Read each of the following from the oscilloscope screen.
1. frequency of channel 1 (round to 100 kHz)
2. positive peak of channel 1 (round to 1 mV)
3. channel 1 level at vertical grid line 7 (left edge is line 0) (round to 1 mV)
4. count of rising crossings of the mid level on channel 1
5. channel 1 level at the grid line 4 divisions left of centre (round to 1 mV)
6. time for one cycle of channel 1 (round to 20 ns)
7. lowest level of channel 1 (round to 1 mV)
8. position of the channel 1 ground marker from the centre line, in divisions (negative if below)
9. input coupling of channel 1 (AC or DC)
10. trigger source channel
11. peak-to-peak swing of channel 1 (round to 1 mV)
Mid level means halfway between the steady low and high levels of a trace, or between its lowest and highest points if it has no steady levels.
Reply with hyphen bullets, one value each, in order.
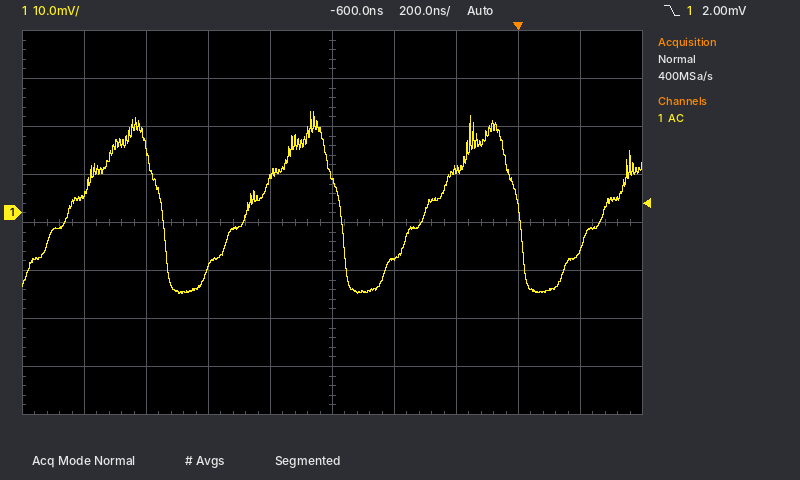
- 1.7 MHz
- 21 mV
- 9 mV
- 4
- 4 mV
- 580 ns
- -17 mV
- +0.2 div
- AC
- channel 1
- 38 mV
